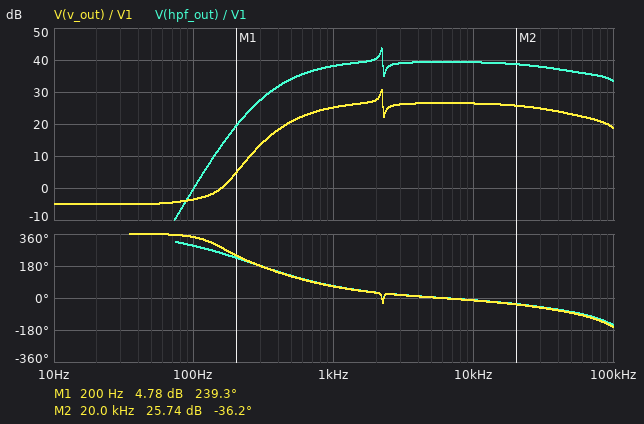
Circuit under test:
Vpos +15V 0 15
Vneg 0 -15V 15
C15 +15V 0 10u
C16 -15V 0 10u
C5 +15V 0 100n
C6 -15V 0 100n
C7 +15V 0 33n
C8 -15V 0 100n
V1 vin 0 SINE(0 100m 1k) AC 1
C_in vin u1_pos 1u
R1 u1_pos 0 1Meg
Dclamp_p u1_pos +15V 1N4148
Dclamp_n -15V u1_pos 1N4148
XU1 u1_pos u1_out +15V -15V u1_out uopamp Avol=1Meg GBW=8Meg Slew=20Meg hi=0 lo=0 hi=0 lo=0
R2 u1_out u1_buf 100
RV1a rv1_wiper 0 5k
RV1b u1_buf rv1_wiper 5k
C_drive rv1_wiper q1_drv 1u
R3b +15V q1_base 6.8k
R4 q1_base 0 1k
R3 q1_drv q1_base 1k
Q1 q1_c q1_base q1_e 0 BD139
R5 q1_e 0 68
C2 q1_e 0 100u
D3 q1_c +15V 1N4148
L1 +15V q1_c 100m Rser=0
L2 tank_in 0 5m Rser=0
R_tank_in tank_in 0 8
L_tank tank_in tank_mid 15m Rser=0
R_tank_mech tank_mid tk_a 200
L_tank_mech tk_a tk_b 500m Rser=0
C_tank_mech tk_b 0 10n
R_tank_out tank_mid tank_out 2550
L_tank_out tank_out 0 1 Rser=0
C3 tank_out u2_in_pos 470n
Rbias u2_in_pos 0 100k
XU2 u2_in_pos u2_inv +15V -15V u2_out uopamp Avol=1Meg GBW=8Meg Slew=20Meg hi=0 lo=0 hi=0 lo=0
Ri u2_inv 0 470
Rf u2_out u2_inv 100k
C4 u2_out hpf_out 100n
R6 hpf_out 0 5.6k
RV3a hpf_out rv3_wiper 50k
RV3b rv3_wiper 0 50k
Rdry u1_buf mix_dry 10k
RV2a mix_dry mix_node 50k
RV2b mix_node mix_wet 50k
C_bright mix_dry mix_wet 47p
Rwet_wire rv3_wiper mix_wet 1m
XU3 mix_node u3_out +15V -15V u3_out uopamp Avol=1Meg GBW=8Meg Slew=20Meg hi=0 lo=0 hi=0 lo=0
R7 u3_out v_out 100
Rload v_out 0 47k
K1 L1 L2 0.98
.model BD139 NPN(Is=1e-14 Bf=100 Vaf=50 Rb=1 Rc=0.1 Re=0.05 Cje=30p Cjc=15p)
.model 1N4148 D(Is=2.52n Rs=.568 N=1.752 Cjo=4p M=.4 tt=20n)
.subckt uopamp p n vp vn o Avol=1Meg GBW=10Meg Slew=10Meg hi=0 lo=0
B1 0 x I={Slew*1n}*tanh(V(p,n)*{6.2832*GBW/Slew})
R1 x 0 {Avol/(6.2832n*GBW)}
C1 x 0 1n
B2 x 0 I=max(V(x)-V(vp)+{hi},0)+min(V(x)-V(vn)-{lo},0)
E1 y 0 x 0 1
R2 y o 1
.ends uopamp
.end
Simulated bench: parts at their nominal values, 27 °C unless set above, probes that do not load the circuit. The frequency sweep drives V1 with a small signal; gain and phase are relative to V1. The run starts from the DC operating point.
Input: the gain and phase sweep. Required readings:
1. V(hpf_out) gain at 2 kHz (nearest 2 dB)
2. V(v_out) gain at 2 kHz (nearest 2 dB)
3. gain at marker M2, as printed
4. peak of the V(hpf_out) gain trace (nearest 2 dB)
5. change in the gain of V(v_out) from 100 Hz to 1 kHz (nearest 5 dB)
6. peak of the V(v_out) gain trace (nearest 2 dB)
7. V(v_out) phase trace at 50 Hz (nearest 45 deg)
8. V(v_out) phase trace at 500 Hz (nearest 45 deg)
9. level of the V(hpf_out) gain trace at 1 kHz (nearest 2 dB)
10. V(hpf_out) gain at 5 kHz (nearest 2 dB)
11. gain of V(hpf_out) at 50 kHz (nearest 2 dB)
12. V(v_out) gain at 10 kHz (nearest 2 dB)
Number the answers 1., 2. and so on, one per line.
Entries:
1. 40 dB
2. 28 dB
3. 25.74 dB
4. 44 dB
5. 30 dB
6. 30 dB
7. 360 deg
8. 135 deg
9. 38 dB
10. 40 dB
11. 36 dB
12. 26 dB
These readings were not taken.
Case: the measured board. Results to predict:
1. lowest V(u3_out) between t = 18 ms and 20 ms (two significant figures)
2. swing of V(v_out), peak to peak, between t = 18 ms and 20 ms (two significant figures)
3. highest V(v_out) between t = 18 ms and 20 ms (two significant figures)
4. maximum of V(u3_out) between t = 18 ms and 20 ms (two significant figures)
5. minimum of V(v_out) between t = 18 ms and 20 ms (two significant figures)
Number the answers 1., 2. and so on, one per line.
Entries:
1. -1.8 V
2. 3.6 V
3. 1.8 V
4. 1.8 V
5. -1.8 V
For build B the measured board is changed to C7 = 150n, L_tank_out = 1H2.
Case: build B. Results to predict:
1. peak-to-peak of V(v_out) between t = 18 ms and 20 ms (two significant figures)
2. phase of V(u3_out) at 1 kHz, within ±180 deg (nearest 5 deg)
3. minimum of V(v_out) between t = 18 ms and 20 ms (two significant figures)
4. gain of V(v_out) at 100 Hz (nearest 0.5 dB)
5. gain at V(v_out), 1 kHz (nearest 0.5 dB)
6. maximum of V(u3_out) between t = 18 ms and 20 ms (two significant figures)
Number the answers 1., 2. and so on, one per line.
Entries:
1. 3.7 V
2. 60 deg
3. -1.9 V
4. -3.5 dB
5. 25.5 dB
6. 1.9 V
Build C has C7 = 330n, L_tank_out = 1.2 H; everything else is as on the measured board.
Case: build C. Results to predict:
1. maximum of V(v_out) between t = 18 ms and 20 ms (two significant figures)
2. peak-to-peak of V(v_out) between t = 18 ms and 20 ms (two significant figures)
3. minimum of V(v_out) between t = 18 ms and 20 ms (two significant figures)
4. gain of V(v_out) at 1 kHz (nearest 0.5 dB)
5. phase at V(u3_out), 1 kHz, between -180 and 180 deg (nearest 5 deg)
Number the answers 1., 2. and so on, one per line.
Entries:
1. 1.9 V
2. 3.7 V
3. -1.9 V
4. 25.5 dB
5. 60 deg
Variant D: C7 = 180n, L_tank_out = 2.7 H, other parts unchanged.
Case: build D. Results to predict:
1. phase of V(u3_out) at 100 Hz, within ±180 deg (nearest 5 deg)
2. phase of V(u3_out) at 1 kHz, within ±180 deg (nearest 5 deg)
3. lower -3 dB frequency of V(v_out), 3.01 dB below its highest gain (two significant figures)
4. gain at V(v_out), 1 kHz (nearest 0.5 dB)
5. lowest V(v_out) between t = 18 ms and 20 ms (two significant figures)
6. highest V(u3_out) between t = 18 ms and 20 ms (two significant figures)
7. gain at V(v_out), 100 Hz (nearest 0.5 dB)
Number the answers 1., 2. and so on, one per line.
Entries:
1. -40 deg
2. 50 deg
3. 2.0 kHz
4. 26.0 dB
5. -2.0 V
6. 2.0 V
7. -2.5 dB
